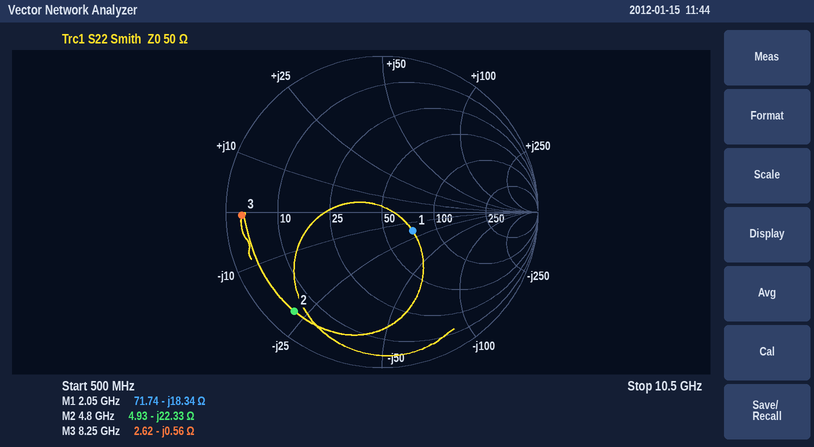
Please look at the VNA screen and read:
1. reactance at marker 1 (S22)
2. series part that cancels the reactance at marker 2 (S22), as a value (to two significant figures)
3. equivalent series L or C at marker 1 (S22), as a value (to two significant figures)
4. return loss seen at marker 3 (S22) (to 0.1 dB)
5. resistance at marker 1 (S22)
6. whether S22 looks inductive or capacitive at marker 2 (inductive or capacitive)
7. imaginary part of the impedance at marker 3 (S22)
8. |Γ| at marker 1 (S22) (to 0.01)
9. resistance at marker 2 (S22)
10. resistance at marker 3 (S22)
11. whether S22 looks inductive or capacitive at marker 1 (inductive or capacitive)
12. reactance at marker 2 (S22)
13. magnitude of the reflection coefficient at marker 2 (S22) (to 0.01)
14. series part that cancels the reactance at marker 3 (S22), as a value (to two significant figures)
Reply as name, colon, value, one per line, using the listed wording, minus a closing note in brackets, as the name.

reactance at marker 1: -18.34 Ω
series part that cancels the reactance at marker 2 (S22), as a value: 740 pH
equivalent series L or C at marker 1 (S22), as a value: 4.2 pF
return loss seen at marker 3 (S22): 0.9 dB
resistance at marker 1: 71.74 Ω
whether S22 looks inductive or capacitive at marker 2: capacitive
imaginary part of the impedance at marker 3: -0.56 Ω
|Γ| at marker 1 (S22): 0.23
resistance at marker 2: 4.93 Ω
resistance at marker 3: 2.62 Ω
whether S22 looks inductive or capacitive at marker 1: capacitive
reactance at marker 2: -22.33 Ω
magnitude of the reflection coefficient at marker 2 (S22): 0.85
series part that cancels the reactance at marker 3 (S22), as a value: 11 pH
